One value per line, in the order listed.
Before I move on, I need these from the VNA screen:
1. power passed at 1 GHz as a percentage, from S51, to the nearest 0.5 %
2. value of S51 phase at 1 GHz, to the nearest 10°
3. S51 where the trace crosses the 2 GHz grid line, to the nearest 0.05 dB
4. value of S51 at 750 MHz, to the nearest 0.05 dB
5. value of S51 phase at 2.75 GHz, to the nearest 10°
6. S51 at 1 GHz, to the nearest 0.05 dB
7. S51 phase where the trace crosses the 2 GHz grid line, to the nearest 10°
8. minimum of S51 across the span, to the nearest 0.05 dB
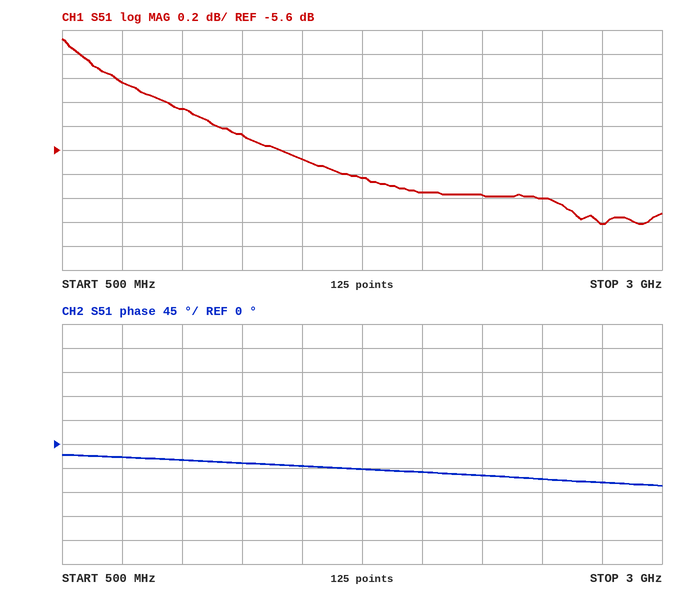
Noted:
30.0 %
-30°
-5.95 dB
-5.05 dB
-70°
-5.25 dB
-50°
-6.20 dB
